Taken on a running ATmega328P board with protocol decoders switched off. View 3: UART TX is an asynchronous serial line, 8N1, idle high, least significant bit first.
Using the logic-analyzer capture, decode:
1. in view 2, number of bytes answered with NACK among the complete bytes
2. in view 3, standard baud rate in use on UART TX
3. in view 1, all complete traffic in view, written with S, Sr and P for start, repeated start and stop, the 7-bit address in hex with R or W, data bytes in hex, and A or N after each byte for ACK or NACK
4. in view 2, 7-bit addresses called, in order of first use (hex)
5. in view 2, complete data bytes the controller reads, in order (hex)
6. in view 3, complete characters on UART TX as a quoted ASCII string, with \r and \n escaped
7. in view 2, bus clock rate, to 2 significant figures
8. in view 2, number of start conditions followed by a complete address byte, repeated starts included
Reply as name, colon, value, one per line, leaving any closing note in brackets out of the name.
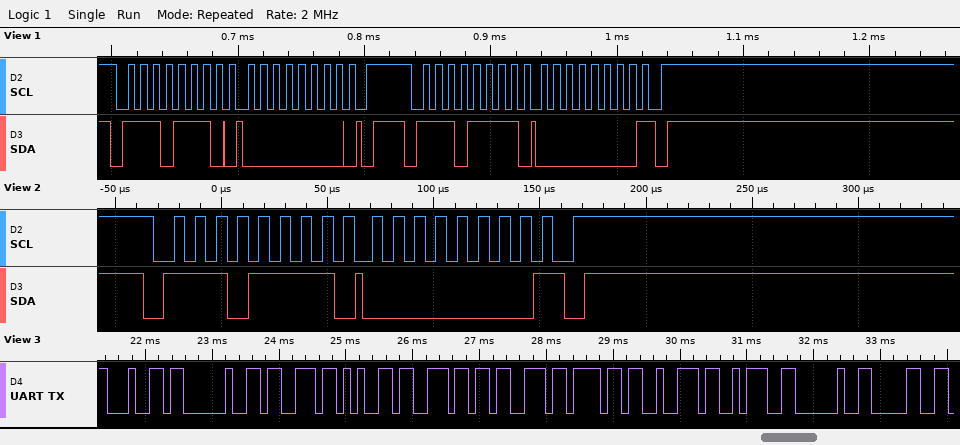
in view 2, number of bytes answered with NACK among the complete bytes: 1
in view 3, standard baud rate in use on UART TX: 9600 baud
in view 1, all complete traffic in view, written with S, Sr and P for start, repeated start and stop, the 7-bit address in hex with R or W, data bytes in hex, and A or N after each byte for ACK or NACK: S 77W A 00 A P S 77R A 00 N P
in view 2, 7-bit addresses called, in order of first use: 0x77
in view 2, complete data bytes the controller reads, in order: 00
in view 3, complete characters on UART TX as a quoted ASCII string, with \r and \n escaped: "d sensor: 0"
in view 2, bus clock rate, to 2 significant figures: 100 kHz
in view 2, number of start conditions followed by a complete address byte, repeated starts included: 1
